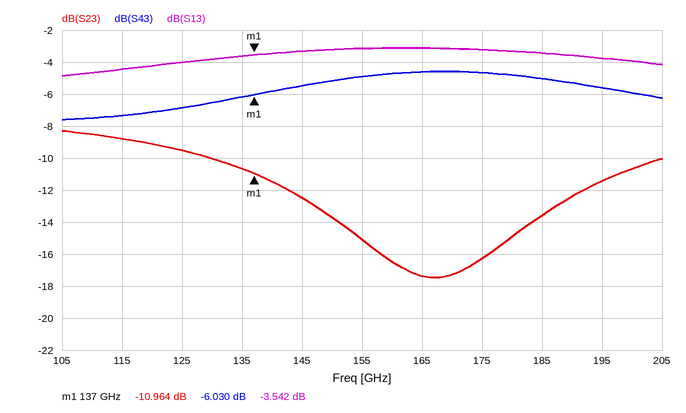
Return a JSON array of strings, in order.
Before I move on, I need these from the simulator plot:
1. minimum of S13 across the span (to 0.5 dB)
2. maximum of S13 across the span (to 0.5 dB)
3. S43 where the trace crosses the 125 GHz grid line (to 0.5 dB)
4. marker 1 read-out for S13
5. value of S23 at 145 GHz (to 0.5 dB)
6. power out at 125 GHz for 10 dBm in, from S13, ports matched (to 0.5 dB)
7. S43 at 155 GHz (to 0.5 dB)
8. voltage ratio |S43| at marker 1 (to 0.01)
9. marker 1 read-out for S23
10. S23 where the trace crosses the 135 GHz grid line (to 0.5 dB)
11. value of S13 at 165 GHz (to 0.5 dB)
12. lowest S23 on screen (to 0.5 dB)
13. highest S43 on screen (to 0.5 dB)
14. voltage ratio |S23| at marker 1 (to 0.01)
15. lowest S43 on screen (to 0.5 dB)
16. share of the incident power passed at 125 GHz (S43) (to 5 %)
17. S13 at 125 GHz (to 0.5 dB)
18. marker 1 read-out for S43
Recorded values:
["-5.0 dB", "-3.0 dB", "-7.0 dB", "-3.542 dB", "-12.5 dB", "6.0 dBm", "-5.0 dB", "0.50", "-10.964 dB", "-10.5 dB", "-3.0 dB", "-17.5 dB", "-4.5 dB", "0.28", "-7.5 dB", "20 %", "-4.0 dB", "-6.030 dB"]
